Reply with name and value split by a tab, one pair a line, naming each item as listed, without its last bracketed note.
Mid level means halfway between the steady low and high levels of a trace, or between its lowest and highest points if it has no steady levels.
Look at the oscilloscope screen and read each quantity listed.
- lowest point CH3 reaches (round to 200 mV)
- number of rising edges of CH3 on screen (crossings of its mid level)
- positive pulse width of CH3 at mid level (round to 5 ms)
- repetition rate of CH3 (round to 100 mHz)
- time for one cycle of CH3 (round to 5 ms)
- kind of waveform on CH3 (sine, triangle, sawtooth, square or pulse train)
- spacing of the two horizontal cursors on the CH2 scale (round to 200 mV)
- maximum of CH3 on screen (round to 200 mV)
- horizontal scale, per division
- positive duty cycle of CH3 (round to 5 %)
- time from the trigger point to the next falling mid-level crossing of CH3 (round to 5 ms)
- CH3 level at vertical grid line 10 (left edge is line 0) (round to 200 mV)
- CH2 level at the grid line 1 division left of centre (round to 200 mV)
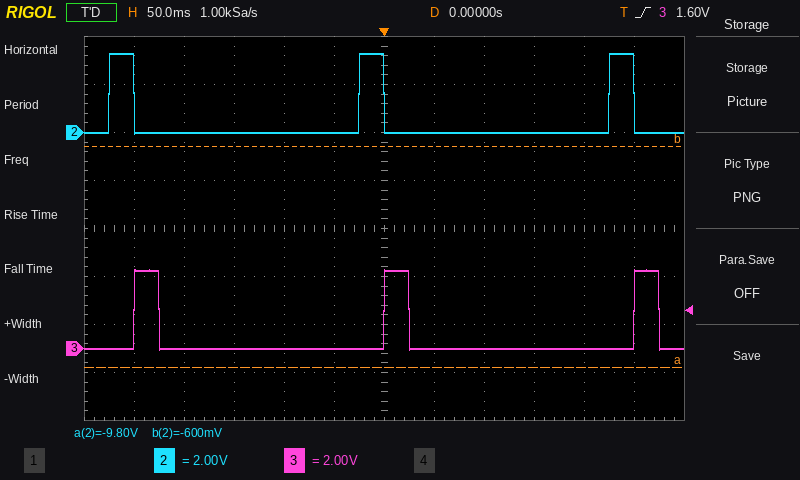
lowest point CH3 reaches	0.0 V
number of rising edges of CH3 on screen	3
positive pulse width of CH3 at mid level	25 ms
repetition rate of CH3	4.0 Hz
time for one cycle of CH3	250 ms
kind of waveform on CH3	pulse train
spacing of the two horizontal cursors on the CH2 scale	9.2 V
maximum of CH3 on screen	3.2 V
horizontal scale, per division	50 ms
positive duty cycle of CH3	10 %
time from the trigger point to the next falling mid-level crossing of CH3	25 ms
CH3 level at vertical grid line 10 (left edge is line 0)	0.0 V
CH2 level at the grid line 1 division left of centre	0.0 V
